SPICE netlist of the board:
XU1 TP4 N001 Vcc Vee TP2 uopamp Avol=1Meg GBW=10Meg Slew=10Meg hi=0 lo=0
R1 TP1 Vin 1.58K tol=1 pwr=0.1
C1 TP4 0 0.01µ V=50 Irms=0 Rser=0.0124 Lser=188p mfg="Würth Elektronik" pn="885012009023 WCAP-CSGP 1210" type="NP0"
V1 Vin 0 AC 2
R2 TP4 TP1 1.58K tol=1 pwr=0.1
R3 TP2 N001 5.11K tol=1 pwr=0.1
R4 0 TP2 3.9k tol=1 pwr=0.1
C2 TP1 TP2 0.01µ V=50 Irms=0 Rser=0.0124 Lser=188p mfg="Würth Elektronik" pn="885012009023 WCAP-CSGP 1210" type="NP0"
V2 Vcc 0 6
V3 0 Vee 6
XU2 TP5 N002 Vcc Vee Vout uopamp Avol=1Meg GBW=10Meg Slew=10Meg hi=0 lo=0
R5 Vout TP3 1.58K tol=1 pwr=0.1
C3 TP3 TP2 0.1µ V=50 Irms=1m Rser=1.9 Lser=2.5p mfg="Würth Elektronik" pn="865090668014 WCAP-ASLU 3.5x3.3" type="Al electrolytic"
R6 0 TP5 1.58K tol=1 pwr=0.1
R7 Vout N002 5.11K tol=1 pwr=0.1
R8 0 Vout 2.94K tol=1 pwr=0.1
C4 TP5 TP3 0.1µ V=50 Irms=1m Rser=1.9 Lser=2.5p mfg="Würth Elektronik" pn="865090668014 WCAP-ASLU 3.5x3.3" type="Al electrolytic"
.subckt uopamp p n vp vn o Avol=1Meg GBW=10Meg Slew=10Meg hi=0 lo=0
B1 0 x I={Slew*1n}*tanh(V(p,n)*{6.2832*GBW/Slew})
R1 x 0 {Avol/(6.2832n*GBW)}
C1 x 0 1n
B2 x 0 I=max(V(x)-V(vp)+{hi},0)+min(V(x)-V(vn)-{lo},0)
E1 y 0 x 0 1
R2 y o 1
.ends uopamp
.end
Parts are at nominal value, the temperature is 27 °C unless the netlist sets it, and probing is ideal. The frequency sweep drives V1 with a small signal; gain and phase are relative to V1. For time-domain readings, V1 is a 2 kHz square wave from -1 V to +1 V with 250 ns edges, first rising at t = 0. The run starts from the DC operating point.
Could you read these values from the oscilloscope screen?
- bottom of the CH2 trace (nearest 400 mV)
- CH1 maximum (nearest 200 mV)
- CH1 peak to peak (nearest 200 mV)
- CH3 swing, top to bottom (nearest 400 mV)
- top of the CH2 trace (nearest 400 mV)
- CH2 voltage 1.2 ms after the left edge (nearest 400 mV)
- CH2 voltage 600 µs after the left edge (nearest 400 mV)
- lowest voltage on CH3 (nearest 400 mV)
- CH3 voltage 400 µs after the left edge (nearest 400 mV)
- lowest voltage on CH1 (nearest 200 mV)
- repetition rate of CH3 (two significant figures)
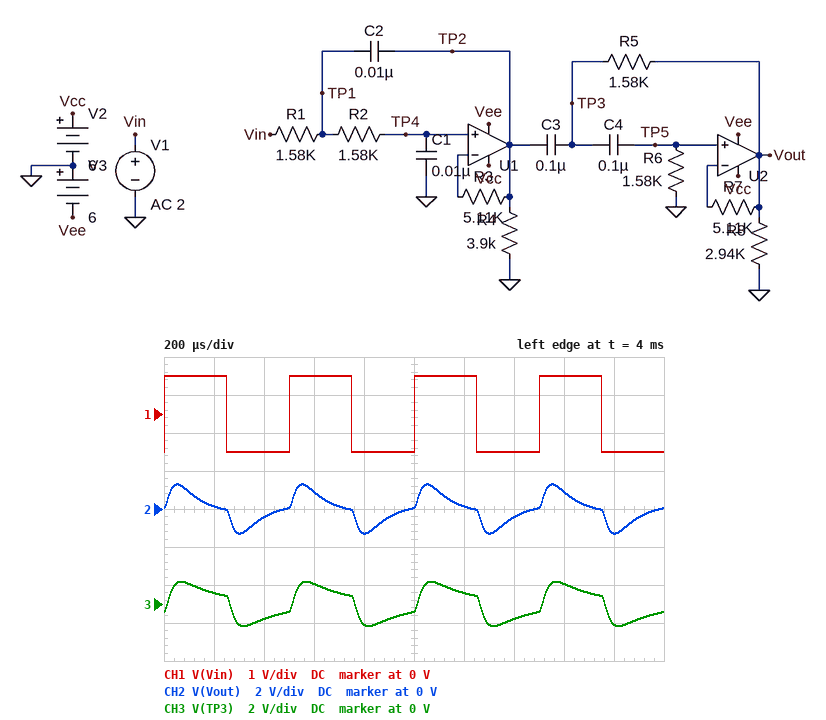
-1.2 V
1.0 V
2.0 V
2.4 V
1.2 V
0 V
800 mV
-1.2 V
-800 mV
-1.0 V
2.0 kHz
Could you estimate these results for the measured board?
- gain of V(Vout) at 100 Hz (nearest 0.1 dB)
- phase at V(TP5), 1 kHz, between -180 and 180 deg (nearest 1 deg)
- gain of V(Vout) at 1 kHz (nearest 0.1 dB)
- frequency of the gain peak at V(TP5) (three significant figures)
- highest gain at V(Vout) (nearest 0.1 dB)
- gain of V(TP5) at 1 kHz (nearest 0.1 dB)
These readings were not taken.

-40.2 dB
79 deg
-6.2 dB
3.18 kHz
-1.7 dB
-6.2 dB
